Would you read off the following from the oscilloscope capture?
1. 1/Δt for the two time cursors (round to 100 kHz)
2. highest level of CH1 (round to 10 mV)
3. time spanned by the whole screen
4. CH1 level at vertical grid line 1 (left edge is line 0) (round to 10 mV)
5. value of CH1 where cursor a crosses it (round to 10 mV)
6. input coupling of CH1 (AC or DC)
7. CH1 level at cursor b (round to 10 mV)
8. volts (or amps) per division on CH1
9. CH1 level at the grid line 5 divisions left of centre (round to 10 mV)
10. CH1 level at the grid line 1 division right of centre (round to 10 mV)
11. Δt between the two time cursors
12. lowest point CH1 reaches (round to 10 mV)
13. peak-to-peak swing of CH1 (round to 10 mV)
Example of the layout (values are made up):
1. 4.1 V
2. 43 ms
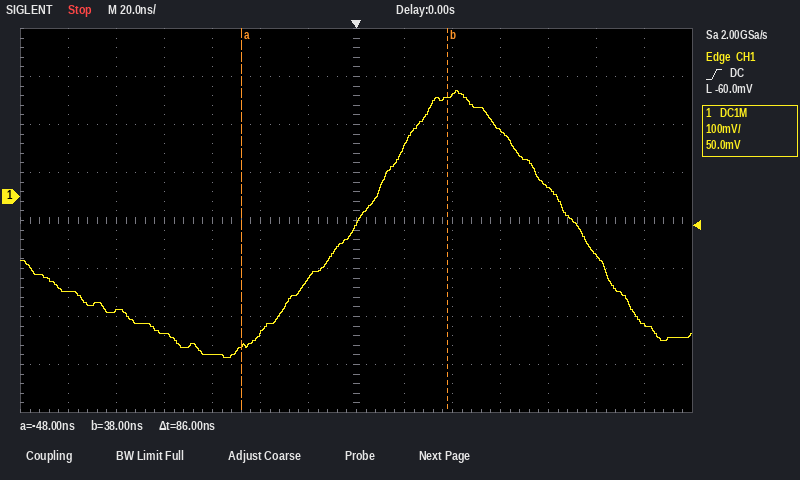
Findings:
1. 11.6 MHz
2. 220 mV
3. 280 ns
4. -200 mV
5. -310 mV
6. DC
7. 210 mV
8. 100 mV
9. -240 mV
10. 100 mV
11. 86 ns
12. -340 mV
13. 560 mV
